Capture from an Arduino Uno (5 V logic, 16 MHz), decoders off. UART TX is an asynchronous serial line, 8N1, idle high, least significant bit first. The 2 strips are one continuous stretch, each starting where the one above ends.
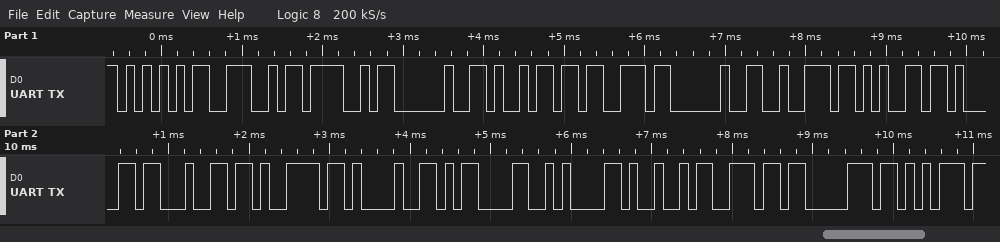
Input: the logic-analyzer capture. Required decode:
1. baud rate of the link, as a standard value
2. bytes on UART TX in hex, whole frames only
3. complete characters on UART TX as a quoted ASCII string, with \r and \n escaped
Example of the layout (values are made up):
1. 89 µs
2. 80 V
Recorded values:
1. 9600 baud
2. 0x55 0x4E 0x4F 0x20 0x69 0x73 0x20 0x72 0x65 0x61 0x64 0x79 0x21 0x0D 0x0A 0x49 0x6E 0x70 0x75
3. "UNO is ready!\r\nInpu"
